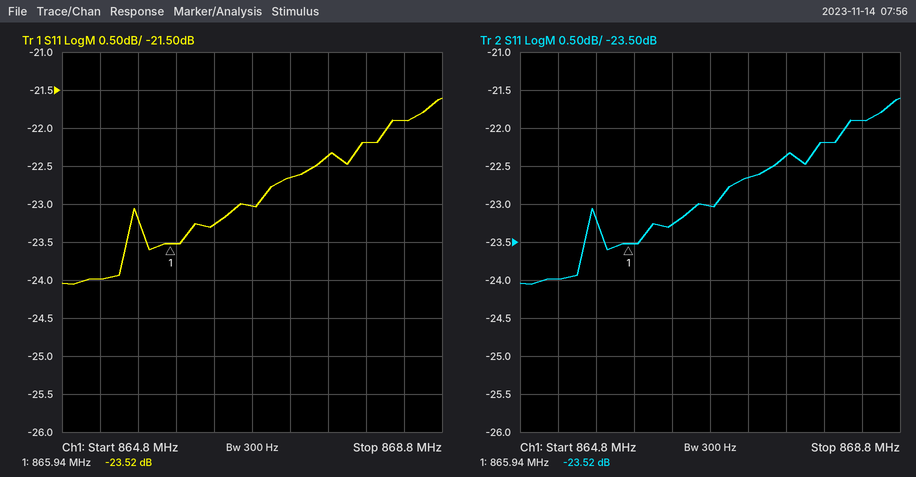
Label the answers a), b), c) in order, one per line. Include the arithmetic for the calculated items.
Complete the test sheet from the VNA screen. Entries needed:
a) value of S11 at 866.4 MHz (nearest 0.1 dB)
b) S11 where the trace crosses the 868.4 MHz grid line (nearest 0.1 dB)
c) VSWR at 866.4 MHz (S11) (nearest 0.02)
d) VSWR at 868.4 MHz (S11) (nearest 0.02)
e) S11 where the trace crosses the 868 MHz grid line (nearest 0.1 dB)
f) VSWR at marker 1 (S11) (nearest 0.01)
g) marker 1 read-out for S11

a) -23.3 dB
b) -21.9 dB
c) |Γ| = 10^(-23.3/20) = 0.0684; VSWR = (1 + 0.0684)/(1 − 0.0684) ≈ 1.15, so 1.14 to the nearest 0.02
d) |Γ| = 10^(-21.9/20) = 0.0804; VSWR = (1 + 0.0804)/(1 − 0.0804) ≈ 1.17, so 1.18 to the nearest 0.02
e) -22.2 dB
f) (1 + 0.0667)/(1 − 0.0667) ≈ 1.14
g) -23.52 dB
